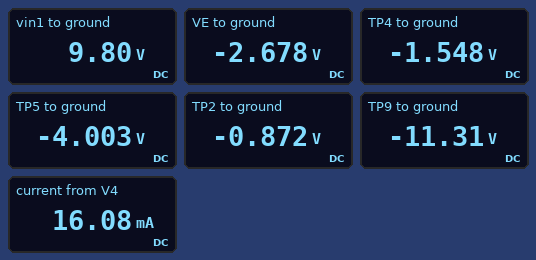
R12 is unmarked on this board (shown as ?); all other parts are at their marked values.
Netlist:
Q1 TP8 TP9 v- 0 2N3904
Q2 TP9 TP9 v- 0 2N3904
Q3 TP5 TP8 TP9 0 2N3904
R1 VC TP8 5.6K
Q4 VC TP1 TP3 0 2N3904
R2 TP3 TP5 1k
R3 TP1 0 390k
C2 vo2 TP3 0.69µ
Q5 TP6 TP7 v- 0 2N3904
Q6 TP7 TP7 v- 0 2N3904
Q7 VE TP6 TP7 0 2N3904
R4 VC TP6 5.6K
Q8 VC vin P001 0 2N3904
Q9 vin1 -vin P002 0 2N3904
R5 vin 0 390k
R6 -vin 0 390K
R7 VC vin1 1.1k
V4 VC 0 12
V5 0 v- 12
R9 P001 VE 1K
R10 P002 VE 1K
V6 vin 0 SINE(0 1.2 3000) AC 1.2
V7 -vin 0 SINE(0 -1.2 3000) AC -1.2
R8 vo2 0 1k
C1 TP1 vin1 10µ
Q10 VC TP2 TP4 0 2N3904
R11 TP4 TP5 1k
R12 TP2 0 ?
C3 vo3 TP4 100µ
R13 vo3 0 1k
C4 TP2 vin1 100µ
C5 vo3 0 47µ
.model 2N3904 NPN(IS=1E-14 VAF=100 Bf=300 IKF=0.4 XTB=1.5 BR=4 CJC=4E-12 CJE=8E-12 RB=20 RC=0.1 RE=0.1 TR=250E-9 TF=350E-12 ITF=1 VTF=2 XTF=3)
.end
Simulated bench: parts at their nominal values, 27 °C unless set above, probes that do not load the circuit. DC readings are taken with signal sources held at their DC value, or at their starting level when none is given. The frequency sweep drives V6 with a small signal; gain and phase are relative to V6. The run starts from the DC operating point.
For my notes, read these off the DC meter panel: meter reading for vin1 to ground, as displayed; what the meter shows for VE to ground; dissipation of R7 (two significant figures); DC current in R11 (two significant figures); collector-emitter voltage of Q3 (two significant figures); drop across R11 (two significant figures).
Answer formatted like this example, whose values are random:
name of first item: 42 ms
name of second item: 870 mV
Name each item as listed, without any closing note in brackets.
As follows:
meter reading for vin1 to ground, as displayed: 9.80 V
what the meter shows for VE to ground: -2.678 V
dissipation of R7: 4.4 mW
DC current in R11: 2.5 mA
collector-emitter voltage of Q3: 7.3 V
drop across R11: 2.5 V
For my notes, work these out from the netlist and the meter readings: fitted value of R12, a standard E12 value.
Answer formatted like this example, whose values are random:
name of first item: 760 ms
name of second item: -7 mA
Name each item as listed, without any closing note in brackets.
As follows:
fitted value of R12, a standard E12 value: 120 kΩ
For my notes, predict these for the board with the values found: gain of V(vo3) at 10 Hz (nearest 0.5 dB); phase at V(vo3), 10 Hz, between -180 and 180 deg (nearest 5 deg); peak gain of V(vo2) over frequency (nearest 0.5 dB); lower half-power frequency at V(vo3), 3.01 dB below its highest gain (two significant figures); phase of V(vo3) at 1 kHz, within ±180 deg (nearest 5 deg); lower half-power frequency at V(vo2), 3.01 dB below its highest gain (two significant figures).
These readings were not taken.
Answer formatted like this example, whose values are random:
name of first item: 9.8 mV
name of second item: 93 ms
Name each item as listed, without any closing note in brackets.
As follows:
gain of V(vo3) at 10 Hz: -2.0 dB
phase at V(vo3), 10 Hz, between -180 and 180 deg: 5 deg
peak gain of V(vo2) over frequency: -1.0 dB
lower half-power frequency at V(vo3), 3.01 dB below its highest gain: 1.1 Hz
phase of V(vo3) at 1 kHz, within ±180 deg: -70 deg
lower half-power frequency at V(vo2), 3.01 dB below its highest gain: 160 Hz
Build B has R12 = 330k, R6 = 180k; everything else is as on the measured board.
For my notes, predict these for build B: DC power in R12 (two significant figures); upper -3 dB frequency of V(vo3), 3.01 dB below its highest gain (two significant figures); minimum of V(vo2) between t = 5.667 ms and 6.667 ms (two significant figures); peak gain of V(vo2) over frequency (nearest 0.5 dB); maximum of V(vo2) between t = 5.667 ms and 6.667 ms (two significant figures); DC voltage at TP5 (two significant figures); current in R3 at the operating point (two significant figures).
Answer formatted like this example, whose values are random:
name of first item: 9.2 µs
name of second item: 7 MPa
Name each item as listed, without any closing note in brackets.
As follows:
DC power in R12: 12 µW
upper -3 dB frequency of V(vo3), 3.01 dB below its highest gain: 320 Hz
minimum of V(vo2) between t = 5.667 ms and 6.667 ms: -950 mV
peak gain of V(vo2) over frequency: -0.5 dB
maximum of V(vo2) between t = 5.667 ms and 6.667 ms: 1.1 V
DC voltage at TP5: -4.8 V
current in R3 at the operating point: 5.6 µA
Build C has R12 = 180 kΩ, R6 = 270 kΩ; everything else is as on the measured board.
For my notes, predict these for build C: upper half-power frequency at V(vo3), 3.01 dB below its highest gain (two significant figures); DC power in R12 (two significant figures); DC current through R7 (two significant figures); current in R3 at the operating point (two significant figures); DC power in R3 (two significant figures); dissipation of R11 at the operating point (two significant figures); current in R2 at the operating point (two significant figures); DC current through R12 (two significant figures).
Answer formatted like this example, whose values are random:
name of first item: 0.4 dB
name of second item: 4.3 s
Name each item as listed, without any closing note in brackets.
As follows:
upper half-power frequency at V(vo3), 3.01 dB below its highest gain: 350 Hz
DC power in R12: 8.6 µW
DC current through R7: 2.0 mA
current in R3 at the operating point: 4.9 µA
DC power in R3: 9.4 µW
dissipation of R11 at the operating point: 5.5 mW
current in R2 at the operating point: 1.7 mA
DC current through R12: 6.9 µA
